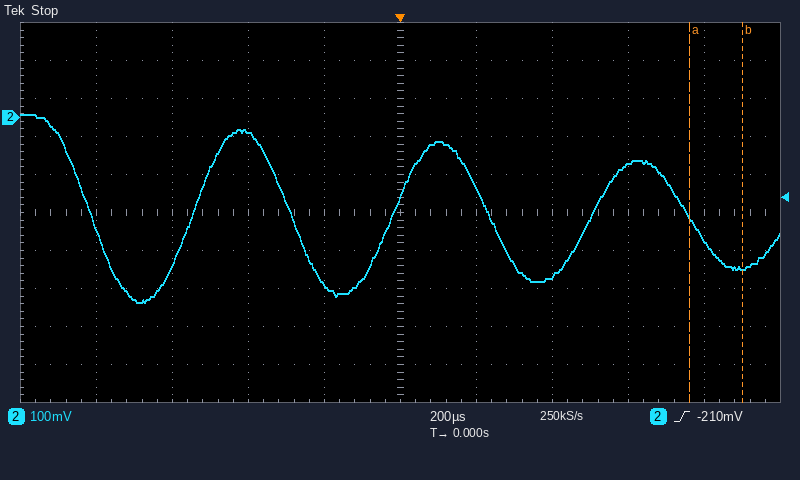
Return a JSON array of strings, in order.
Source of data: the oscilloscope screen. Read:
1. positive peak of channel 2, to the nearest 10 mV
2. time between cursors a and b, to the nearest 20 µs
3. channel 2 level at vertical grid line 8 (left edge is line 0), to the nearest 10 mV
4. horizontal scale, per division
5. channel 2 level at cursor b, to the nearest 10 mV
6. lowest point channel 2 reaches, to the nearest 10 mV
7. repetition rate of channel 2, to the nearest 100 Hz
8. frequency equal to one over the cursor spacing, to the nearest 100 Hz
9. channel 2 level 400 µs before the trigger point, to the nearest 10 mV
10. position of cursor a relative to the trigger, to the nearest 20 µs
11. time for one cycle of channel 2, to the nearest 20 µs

["10 mV", "140 µs", "-120 mV", "200 µs", "-400 mV", "-490 mV", "1.9 kHz", "7.1 kHz", "-40 mV", "+760 µs", "520 µs"]
